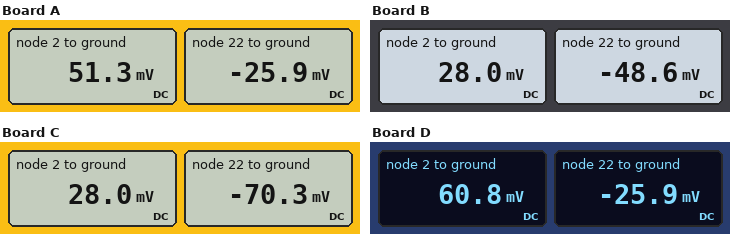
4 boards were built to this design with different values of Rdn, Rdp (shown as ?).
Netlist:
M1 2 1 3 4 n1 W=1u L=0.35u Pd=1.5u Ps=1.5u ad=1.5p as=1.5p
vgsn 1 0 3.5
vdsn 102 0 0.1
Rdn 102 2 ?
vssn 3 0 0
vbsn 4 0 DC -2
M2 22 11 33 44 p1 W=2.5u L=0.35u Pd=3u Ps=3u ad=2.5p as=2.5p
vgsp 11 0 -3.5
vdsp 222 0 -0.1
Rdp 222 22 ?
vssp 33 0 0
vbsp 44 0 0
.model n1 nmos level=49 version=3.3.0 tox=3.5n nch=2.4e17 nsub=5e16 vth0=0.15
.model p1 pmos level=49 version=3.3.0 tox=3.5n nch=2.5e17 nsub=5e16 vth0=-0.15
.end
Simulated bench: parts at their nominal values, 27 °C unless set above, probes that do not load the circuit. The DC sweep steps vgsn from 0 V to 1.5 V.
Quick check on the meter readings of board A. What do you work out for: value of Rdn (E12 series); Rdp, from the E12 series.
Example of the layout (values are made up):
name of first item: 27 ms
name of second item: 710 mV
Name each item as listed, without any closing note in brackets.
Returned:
value of Rdn: 820 Ω
Rdp, from the E12 series: 2.2 kΩ
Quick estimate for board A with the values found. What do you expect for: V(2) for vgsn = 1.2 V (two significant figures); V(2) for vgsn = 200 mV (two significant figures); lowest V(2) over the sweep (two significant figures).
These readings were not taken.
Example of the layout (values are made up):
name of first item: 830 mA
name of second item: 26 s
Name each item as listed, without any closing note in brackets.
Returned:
V(2) for vgsn = 1.2 V: 75 mV
V(2) for vgsn = 200 mV: 100 mV
lowest V(2) over the sweep: 68 mV
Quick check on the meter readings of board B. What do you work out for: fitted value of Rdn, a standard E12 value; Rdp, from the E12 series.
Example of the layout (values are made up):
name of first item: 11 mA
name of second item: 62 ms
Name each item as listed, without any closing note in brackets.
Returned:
fitted value of Rdn, a standard E12 value: 2.2 kΩ
Rdp, from the E12 series: 820 Ω
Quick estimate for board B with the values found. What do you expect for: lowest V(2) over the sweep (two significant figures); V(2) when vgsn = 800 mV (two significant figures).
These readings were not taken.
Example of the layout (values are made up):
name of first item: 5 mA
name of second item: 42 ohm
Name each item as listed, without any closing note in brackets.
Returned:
lowest V(2) over the sweep: 43 mV
V(2) when vgsn = 800 mV: 79 mV
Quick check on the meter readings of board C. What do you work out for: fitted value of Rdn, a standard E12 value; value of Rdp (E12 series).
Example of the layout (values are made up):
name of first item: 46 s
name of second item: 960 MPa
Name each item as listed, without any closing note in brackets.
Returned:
fitted value of Rdn, a standard E12 value: 2.2 kΩ
value of Rdp: 330 Ω
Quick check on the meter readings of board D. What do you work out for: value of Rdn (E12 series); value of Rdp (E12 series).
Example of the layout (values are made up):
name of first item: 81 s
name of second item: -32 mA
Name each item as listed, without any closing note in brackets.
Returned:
value of Rdn: 560 Ω
value of Rdp: 2.2 kΩ
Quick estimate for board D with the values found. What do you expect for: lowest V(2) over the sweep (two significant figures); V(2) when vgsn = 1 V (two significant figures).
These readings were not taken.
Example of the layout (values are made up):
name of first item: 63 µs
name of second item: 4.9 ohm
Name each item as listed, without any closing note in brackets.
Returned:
lowest V(2) over the sweep: 76 mV
V(2) when vgsn = 1 V: 87 mV
